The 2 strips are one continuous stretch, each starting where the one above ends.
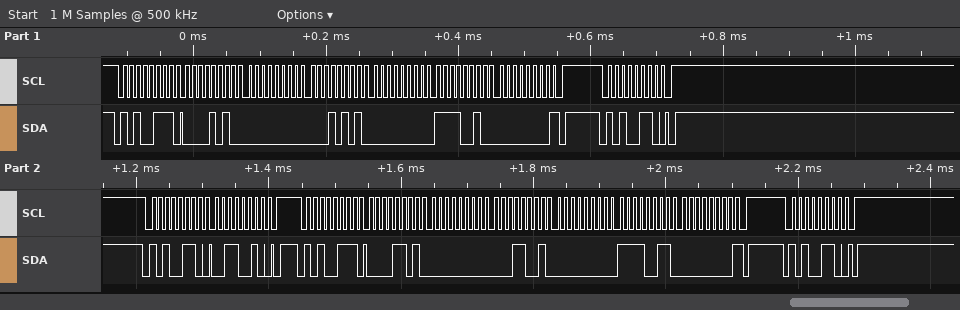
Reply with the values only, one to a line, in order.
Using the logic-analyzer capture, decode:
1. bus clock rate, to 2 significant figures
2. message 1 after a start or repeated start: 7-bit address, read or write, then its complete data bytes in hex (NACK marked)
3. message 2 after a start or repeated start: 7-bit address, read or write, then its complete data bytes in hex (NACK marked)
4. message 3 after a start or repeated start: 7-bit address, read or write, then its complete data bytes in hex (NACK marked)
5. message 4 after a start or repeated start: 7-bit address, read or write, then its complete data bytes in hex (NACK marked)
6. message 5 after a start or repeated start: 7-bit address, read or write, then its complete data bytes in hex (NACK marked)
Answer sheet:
100 kHz
0x53 read: 0A 00 15 00 F2 00 NACK
0x53 write
0x53 write: 32
0x53 read: 0D 00 19 00 F3 00 NACK
0x53 write
